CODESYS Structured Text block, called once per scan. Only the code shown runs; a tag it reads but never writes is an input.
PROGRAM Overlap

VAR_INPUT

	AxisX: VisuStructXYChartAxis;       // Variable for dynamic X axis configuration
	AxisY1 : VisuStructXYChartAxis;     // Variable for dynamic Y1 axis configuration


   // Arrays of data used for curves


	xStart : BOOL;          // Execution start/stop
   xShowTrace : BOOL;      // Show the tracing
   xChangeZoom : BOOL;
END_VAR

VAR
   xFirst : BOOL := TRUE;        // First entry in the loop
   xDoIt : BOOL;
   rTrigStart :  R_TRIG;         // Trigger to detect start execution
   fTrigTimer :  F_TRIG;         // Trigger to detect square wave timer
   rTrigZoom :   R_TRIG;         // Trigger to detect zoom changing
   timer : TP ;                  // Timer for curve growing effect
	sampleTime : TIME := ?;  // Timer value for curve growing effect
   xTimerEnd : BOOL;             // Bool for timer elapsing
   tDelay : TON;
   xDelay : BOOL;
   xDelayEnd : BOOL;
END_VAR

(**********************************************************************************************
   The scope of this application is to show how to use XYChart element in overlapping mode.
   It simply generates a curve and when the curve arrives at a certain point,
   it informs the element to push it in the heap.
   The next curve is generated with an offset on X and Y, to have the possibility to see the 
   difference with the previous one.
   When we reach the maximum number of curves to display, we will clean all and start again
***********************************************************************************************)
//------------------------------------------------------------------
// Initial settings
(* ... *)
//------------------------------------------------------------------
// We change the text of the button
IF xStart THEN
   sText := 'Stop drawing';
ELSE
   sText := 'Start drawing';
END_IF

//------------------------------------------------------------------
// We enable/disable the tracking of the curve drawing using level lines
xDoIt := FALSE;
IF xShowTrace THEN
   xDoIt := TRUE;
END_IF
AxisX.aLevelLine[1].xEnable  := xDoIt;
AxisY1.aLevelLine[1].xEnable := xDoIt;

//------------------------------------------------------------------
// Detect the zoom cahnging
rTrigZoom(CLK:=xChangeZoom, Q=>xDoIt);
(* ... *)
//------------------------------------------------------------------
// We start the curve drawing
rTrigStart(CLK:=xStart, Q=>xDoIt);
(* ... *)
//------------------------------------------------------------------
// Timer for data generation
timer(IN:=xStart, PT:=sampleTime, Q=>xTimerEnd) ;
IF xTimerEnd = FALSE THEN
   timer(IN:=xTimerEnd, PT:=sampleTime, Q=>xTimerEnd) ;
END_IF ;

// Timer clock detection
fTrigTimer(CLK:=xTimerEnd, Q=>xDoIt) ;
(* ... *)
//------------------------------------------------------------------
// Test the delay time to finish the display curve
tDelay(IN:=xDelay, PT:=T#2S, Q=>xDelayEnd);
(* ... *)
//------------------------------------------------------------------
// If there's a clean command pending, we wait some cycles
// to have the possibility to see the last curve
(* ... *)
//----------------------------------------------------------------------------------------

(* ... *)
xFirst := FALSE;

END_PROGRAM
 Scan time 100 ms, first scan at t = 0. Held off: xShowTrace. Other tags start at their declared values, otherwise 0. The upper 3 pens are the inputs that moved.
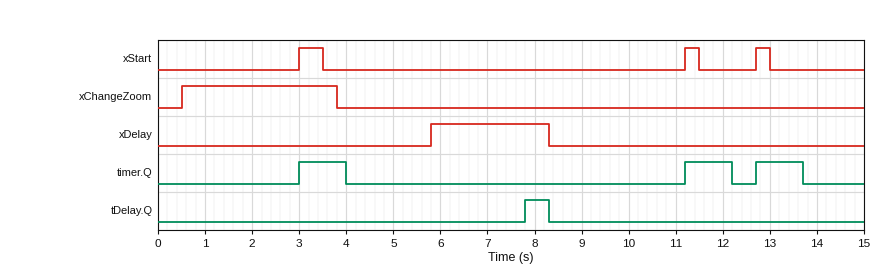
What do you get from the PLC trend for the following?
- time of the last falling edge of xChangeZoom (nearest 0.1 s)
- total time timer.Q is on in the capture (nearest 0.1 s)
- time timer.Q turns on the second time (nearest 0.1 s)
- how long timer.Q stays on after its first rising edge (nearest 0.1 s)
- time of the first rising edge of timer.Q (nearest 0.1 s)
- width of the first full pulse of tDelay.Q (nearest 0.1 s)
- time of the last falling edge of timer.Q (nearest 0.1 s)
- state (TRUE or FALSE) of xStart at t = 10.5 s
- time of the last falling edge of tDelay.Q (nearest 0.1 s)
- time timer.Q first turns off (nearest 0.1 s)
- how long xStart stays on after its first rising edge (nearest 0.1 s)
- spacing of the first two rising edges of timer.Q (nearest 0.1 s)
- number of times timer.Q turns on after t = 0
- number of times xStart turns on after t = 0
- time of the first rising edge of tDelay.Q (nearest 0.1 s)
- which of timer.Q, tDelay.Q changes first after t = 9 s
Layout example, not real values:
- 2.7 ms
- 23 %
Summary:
- 3.8 s
- 3.0 s
- 11.2 s
- 1.0 s
- 3.0 s
- 0.5 s
- 13.7 s
- FALSE
- 8.3 s
- 4.0 s
- 0.5 s
- 8.2 s
- 3
- 3
- 7.8 s
- timer.Q
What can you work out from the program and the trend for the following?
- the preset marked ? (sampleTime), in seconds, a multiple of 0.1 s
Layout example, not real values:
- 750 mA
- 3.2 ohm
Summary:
- 1.0 s
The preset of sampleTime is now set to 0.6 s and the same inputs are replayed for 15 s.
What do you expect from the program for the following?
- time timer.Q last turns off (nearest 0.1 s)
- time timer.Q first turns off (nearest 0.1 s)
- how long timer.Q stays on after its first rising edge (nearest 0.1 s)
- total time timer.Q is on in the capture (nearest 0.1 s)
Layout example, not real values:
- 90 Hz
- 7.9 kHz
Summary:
- 13.3 s
- 3.6 s
- 0.6 s
- 1.8 s
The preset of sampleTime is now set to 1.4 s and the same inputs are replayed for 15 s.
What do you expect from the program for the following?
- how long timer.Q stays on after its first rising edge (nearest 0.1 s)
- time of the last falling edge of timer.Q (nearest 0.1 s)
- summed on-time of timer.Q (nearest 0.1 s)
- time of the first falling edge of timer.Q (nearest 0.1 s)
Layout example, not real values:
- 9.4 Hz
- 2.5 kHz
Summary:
- 1.4 s
- 14.1 s
- 4.2 s
- 4.4 s
